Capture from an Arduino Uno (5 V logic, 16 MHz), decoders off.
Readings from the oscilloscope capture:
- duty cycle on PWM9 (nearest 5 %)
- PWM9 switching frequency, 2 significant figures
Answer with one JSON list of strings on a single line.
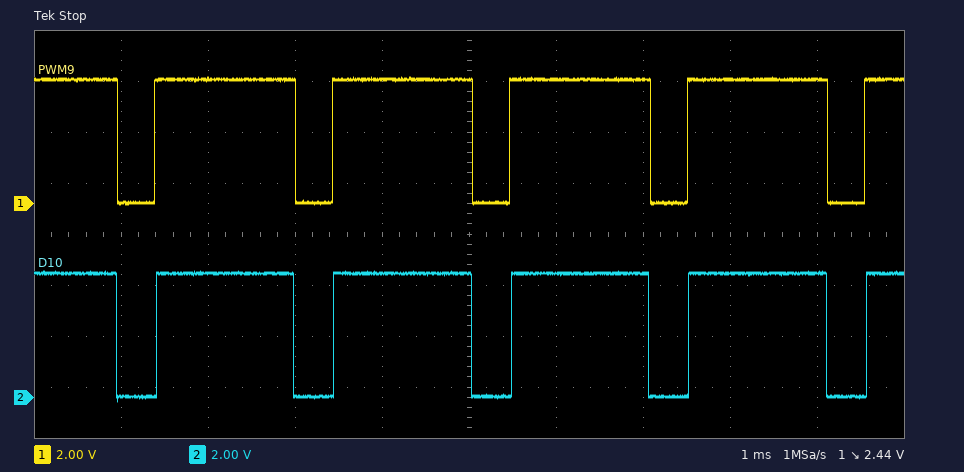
["80 %", "490 Hz"]
